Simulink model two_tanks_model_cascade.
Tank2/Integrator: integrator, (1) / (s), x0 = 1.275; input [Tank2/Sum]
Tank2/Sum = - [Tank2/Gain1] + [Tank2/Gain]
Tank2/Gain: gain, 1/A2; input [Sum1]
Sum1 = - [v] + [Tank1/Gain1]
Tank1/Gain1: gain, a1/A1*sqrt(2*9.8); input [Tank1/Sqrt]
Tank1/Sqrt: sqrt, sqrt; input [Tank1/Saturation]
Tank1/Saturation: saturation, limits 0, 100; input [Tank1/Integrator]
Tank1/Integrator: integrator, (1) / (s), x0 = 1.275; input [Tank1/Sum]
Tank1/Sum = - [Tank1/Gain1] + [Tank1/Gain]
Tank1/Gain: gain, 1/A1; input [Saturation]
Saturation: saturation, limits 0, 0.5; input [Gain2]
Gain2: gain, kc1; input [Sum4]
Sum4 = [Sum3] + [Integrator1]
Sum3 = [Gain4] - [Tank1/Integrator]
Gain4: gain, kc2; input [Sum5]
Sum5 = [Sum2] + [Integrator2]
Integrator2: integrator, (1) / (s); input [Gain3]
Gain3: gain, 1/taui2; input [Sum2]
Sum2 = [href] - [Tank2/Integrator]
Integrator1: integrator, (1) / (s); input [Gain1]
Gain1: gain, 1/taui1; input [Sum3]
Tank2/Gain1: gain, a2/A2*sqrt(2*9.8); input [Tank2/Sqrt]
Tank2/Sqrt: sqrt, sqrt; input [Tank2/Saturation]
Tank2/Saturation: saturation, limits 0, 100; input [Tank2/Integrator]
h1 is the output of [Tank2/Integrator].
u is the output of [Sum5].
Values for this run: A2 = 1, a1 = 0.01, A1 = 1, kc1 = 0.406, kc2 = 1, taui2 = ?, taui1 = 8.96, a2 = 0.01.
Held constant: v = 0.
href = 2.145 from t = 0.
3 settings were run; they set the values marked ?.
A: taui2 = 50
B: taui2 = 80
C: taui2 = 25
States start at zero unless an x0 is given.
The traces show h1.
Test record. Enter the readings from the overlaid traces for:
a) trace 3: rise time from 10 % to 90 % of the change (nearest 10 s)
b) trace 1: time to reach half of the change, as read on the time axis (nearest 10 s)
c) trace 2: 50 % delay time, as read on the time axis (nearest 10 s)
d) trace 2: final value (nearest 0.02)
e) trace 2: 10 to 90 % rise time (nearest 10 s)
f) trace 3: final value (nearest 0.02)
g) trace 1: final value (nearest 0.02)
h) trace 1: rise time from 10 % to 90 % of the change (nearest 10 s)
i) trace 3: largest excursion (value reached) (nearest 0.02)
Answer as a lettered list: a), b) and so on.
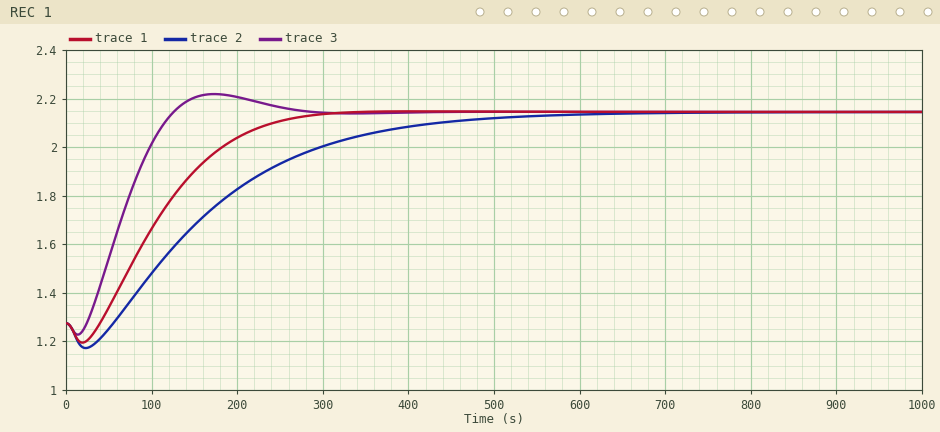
a) 70 s
b) 110 s
c) 160 s
d) 2.14
e) 280 s
f) 2.14
g) 2.14
h) 160 s
i) 2.22
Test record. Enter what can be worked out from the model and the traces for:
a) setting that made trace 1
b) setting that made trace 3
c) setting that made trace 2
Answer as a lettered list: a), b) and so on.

a) A
b) C
c) B
